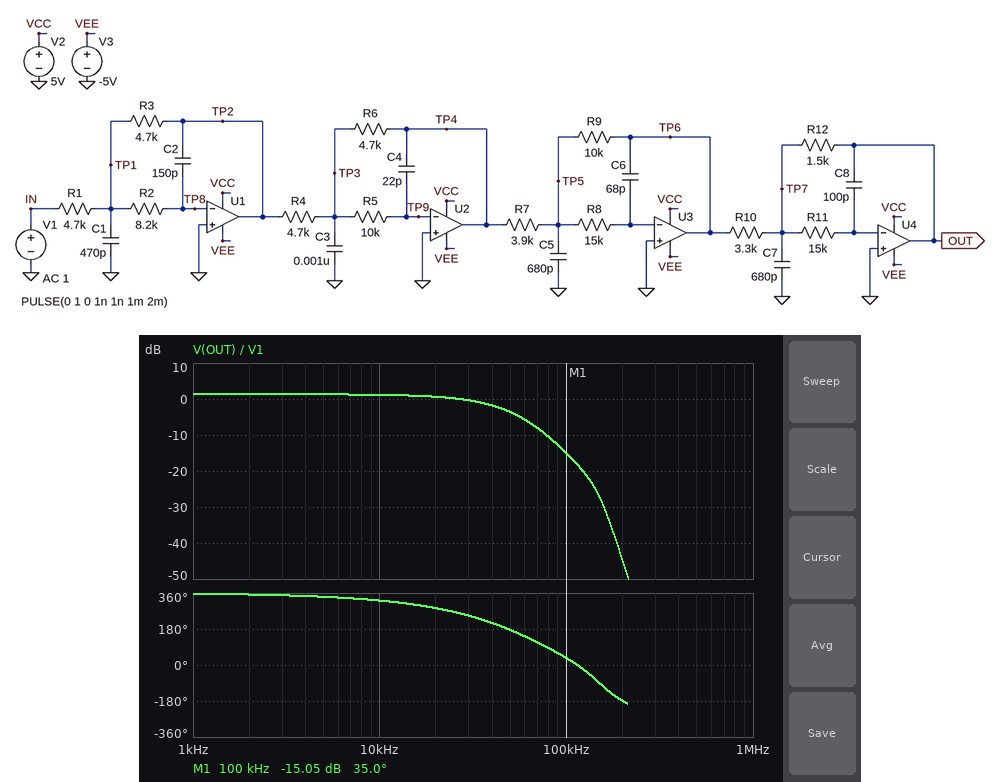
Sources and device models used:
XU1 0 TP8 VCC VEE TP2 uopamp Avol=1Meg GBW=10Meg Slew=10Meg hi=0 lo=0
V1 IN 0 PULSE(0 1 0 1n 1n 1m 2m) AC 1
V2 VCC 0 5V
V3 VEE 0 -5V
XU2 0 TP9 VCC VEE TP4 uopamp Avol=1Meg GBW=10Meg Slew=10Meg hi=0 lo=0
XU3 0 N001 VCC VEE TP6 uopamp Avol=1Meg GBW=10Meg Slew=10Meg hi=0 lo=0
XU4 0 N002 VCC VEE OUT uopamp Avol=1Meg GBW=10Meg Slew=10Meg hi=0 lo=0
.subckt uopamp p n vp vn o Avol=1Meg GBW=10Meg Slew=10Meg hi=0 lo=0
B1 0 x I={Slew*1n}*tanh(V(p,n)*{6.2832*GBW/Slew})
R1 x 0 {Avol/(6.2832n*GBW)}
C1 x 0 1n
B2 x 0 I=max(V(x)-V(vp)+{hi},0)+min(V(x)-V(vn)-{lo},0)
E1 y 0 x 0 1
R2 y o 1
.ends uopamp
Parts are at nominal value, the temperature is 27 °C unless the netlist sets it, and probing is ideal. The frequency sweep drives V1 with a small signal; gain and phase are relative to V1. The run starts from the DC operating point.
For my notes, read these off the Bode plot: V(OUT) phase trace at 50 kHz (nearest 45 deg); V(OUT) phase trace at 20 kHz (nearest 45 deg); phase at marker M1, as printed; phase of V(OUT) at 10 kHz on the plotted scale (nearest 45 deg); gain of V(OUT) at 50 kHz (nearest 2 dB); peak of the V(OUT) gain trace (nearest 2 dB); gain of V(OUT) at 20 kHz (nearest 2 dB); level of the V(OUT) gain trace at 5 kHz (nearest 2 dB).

180 deg
270 deg
35.0 deg
315 deg
-4 dB
2 dB
0 dB
2 dB
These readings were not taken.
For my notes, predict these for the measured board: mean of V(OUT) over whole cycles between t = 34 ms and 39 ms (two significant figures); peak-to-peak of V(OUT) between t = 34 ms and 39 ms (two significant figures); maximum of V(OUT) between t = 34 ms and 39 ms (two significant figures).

580 mV
1.2 V
1.2 V
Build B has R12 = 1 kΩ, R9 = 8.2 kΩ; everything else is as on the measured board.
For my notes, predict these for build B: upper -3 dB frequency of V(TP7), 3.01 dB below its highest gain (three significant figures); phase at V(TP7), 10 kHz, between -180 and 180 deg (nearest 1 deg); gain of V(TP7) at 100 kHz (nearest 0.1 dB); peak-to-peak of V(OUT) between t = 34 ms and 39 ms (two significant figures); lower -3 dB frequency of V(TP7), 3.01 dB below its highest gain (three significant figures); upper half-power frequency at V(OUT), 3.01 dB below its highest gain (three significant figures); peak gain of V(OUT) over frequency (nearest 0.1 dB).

89.8 kHz
-125 deg
-18.4 dB
650 mV
25.0 kHz
44.6 kHz
-3.9 dB
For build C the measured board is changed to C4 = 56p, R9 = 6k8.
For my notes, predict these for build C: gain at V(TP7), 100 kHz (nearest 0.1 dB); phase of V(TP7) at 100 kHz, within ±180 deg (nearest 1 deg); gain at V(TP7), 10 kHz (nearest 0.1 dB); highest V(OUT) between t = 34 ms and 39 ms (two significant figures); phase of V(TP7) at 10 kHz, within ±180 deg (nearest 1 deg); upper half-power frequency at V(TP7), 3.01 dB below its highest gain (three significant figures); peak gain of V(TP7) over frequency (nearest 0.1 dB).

-18.1 dB
-107 deg
-22.5 dB
820 mV
-127 deg
84.7 kHz
-11.1 dB
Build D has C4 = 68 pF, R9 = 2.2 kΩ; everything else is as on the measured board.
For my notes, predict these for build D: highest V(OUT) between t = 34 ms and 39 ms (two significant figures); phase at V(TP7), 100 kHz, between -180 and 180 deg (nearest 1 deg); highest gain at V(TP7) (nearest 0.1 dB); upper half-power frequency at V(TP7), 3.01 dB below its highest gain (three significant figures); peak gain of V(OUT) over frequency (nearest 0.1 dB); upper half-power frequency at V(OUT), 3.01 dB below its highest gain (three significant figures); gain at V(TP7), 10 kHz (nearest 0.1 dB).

270 mV
-75 deg
-19.2 dB
91.8 kHz
-11.8 dB
63.2 kHz
-32.3 dB
